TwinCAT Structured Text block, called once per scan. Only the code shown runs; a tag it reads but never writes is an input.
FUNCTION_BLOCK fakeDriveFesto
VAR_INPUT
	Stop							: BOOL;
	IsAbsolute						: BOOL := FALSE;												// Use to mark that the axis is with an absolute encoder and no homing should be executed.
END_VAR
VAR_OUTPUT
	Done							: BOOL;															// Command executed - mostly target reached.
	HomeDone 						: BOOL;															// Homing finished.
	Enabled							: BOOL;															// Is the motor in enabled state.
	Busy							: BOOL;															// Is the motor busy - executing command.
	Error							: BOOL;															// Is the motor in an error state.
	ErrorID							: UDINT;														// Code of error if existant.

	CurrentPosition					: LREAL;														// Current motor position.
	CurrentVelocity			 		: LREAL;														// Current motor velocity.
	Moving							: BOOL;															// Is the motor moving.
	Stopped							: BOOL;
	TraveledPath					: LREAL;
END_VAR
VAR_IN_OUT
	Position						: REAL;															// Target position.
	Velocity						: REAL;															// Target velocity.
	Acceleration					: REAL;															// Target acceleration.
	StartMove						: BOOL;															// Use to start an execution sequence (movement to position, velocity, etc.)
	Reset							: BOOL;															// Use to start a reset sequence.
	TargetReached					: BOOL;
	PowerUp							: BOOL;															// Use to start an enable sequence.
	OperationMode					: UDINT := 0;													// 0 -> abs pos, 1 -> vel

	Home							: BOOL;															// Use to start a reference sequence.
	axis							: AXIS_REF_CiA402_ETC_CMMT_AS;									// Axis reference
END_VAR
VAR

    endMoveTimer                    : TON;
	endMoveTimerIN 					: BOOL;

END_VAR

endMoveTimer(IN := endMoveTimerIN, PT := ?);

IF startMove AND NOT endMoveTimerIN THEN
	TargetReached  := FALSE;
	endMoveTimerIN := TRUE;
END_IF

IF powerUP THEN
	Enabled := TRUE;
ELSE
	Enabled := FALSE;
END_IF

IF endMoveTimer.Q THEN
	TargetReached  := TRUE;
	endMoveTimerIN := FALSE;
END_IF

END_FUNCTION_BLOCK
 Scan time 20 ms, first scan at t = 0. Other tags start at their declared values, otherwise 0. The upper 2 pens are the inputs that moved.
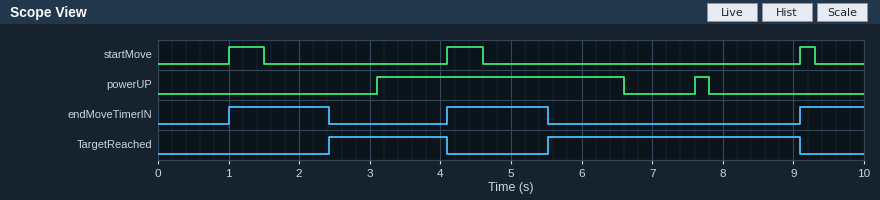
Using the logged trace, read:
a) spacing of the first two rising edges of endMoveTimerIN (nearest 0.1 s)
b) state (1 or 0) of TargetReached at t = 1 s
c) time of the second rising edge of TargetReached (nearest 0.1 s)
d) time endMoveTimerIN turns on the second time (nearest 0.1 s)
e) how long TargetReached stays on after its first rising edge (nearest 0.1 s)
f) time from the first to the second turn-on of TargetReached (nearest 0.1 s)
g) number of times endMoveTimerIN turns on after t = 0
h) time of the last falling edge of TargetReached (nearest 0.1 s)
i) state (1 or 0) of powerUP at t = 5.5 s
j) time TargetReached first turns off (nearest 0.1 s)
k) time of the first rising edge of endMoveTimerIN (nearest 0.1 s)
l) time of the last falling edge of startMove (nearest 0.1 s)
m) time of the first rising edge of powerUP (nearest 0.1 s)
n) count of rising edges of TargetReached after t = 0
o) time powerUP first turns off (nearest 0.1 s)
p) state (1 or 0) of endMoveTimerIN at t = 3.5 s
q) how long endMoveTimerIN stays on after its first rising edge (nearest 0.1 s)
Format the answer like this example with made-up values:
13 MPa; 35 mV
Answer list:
3.1 s; 0; 5.5 s; 4.1 s; 1.7 s; 3.1 s; 3; 9.1 s; 1; 4.1 s; 1.0 s; 9.3 s; 3.1 s; 2; 6.6 s; 0; 1.4 s
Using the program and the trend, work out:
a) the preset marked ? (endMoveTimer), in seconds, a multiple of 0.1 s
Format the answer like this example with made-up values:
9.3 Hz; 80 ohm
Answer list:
1.4 s
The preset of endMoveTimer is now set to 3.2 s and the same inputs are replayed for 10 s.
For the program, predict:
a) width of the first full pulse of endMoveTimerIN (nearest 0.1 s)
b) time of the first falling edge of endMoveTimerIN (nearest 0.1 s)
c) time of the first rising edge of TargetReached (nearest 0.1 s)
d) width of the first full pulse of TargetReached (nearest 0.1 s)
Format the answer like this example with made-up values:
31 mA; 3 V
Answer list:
3.2 s; 4.2 s; 4.2 s; 0.0 s
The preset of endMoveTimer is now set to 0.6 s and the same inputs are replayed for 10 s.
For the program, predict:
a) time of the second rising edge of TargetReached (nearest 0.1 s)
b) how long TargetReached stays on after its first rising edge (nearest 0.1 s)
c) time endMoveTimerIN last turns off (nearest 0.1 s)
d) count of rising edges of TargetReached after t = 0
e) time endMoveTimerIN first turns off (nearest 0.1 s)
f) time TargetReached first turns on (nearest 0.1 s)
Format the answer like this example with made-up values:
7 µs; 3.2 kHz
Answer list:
4.7 s; 2.5 s; 9.7 s; 3; 1.6 s; 1.6 s
